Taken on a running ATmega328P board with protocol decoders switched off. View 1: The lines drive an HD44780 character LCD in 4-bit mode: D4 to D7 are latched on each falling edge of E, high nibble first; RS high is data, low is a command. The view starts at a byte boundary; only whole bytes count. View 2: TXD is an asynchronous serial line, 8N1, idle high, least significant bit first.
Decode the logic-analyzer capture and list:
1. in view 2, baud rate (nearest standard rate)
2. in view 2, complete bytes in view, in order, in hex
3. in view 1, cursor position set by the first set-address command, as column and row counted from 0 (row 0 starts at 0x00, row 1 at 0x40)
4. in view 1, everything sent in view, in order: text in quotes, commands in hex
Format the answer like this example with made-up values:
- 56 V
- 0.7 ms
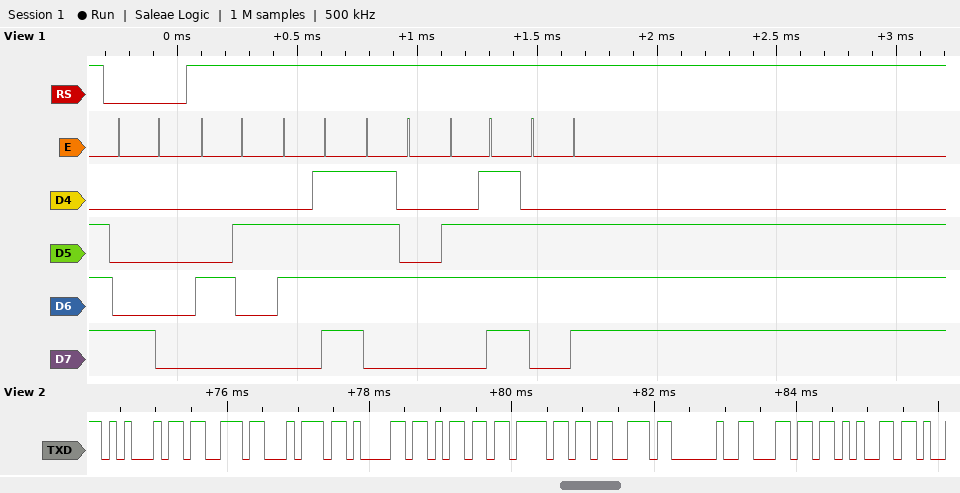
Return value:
- 9600 baud
- 45 73 74 61 6D 6F 73 20 6C 65
- column 0, row 0
- 0x80 "Boton"
